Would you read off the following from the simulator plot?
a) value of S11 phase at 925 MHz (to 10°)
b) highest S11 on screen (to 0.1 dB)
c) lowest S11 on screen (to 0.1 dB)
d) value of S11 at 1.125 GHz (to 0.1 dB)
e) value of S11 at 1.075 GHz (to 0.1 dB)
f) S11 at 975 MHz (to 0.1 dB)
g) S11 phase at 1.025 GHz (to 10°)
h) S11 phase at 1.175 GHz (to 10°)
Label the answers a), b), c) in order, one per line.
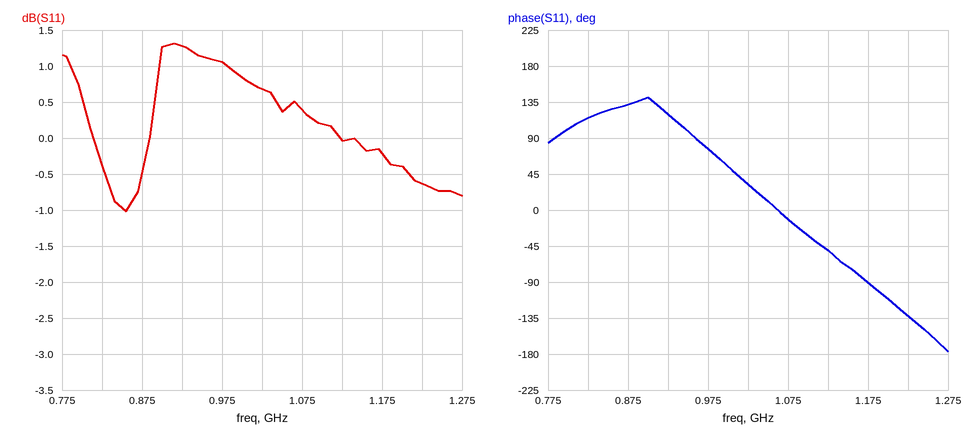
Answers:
a) 120°
b) 1.3 dB
c) -1.0 dB
d) 0.0 dB
e) 0.4 dB
f) 1.1 dB
g) 30°
h) -90°
